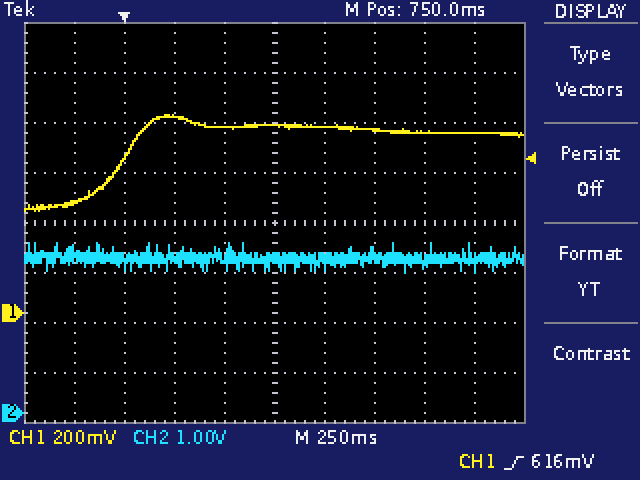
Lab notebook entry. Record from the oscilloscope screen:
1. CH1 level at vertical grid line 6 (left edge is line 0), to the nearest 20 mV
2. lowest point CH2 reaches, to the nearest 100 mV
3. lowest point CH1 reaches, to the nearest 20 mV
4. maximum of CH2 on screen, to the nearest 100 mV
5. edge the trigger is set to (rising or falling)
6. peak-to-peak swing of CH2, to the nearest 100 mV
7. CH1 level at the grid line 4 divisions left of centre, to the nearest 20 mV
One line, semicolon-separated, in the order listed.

740 mV; 2.8 V; 400 mV; 3.4 V; rising; 600 mV; 440 mV
